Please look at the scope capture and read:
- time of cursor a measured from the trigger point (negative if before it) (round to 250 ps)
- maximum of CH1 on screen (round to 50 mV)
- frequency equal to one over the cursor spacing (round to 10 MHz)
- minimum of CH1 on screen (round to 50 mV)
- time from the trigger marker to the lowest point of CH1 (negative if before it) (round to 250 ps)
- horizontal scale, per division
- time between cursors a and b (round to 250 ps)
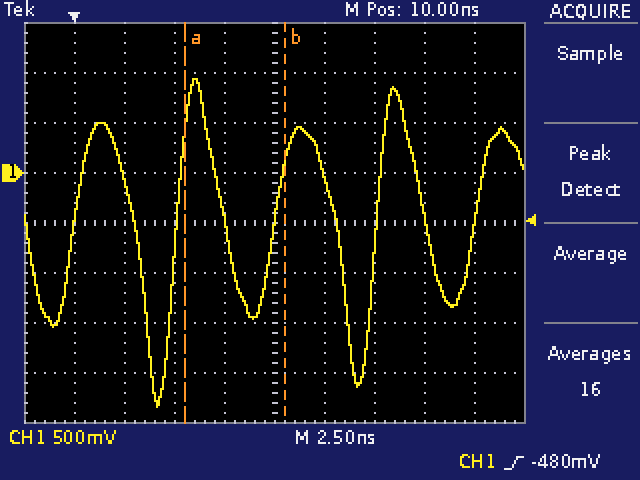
+5.50 ns
950 mV
200 MHz
-2.35 V
+4.25 ns
2.5 ns
5.00 ns
